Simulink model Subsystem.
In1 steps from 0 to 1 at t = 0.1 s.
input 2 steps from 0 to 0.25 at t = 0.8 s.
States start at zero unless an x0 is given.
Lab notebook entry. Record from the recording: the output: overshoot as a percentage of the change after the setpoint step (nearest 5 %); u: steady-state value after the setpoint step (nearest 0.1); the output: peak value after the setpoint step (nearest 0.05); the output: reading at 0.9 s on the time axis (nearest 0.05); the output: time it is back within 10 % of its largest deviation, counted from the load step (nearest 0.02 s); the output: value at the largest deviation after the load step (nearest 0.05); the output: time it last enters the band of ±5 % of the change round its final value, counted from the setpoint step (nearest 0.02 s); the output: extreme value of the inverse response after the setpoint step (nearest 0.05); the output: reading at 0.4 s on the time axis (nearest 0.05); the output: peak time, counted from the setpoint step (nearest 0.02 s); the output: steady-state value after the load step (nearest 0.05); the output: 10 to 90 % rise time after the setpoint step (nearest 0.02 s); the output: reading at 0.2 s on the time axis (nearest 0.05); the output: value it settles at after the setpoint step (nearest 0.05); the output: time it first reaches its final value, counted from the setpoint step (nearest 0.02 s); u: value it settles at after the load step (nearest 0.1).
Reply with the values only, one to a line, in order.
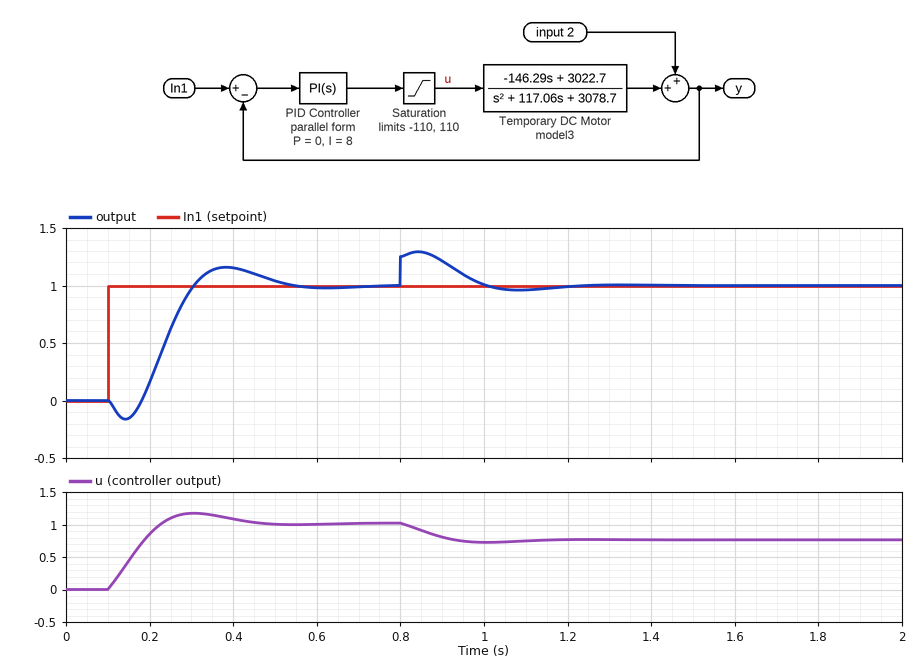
15 %
1.0
1.15
1.20
0.34 s
1.30
0.40 s
-0.15
1.15
0.28 s
1.00
0.10 s
0.15
1.00
0.20 s
0.8
